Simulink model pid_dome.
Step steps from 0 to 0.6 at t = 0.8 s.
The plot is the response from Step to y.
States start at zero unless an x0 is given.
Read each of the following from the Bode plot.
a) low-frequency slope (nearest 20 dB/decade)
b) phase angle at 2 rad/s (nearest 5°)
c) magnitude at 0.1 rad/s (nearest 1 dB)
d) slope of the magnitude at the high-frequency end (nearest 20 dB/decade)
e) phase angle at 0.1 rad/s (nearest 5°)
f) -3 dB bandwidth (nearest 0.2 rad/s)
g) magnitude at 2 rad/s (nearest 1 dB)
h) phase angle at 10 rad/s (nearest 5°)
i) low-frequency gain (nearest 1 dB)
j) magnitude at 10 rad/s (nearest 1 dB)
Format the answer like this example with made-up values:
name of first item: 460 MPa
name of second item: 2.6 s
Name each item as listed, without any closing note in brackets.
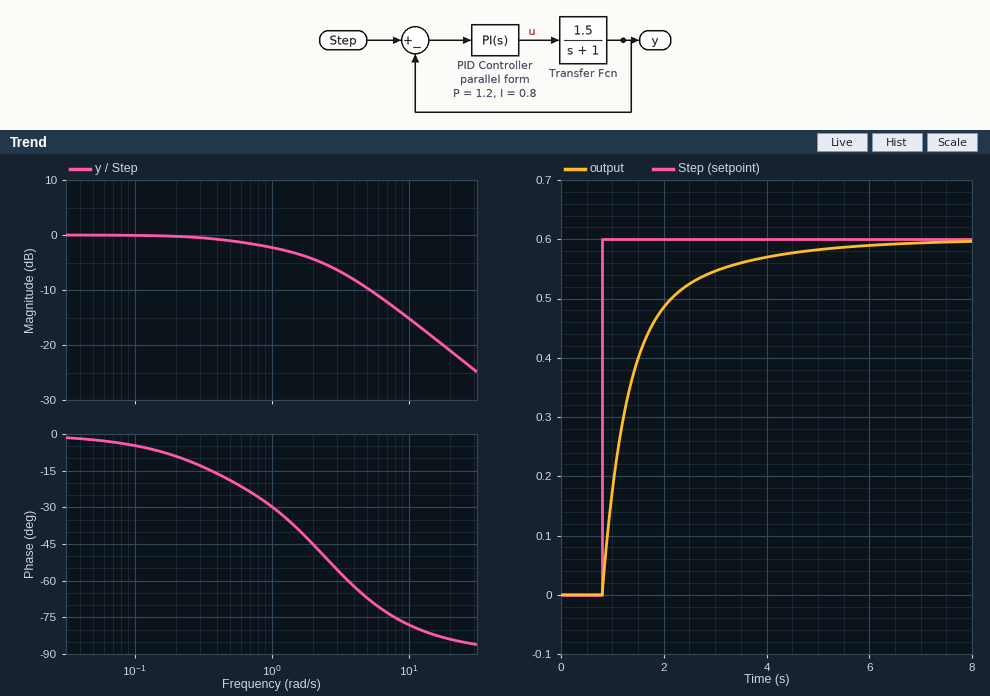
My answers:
low-frequency slope: 0 dB/decade
phase angle at 2 rad/s: -45°
magnitude at 0.1 rad/s: 0 dB
slope of the magnitude at the high-frequency end: -20 dB/decade
phase angle at 0.1 rad/s: -5°
-3 dB bandwidth: 1.4 rad/s
magnitude at 2 rad/s: -4 dB
phase angle at 10 rad/s: -80°
low-frequency gain: 0 dB
magnitude at 10 rad/s: -15 dB
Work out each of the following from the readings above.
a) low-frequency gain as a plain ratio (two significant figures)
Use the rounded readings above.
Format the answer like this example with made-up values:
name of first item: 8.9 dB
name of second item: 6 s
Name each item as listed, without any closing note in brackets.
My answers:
low-frequency gain as a plain ratio: 1.0
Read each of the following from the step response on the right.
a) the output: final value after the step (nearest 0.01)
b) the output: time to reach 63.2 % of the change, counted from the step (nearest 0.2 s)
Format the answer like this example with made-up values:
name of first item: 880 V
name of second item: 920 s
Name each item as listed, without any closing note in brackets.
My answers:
the output: final value after the step: 0.60
the output: time to reach 63.2 % of the change, counted from the step: 0.6 s
